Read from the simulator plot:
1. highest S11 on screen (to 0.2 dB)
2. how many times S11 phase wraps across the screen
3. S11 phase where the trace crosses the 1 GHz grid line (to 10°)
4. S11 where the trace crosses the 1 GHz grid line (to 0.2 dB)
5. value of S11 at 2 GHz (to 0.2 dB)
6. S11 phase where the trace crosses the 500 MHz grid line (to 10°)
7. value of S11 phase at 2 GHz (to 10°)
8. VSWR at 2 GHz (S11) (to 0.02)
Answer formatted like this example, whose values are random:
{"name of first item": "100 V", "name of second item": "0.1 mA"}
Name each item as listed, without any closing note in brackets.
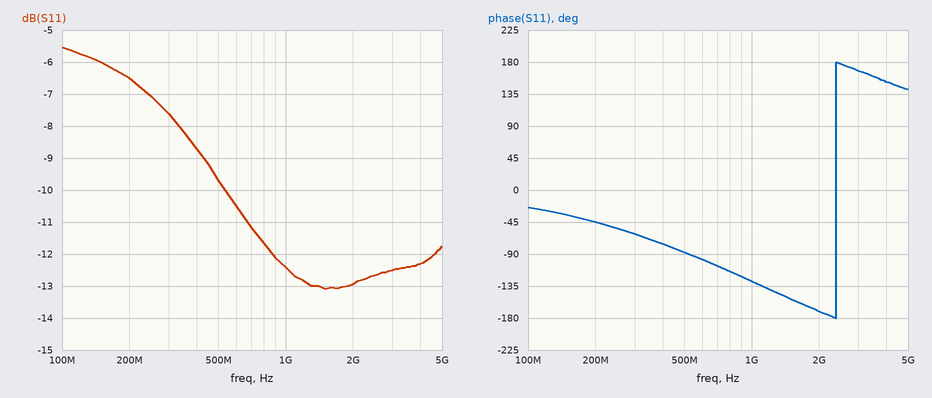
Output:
{"highest S11 on screen": "-5.6 dB", "how many times S11 phase wraps across the screen": "1", "S11 phase where the trace crosses the 1 GHz grid line": "-130°", "S11 where the trace crosses the 1 GHz grid line": "-12.4 dB", "value of S11 at 2 GHz": "-13.0 dB", "S11 phase where the trace crosses the 500 MHz grid line": "-90°", "value of S11 phase at 2 GHz": "-170°", "VSWR at 2 GHz (S11)": "1.58"}
